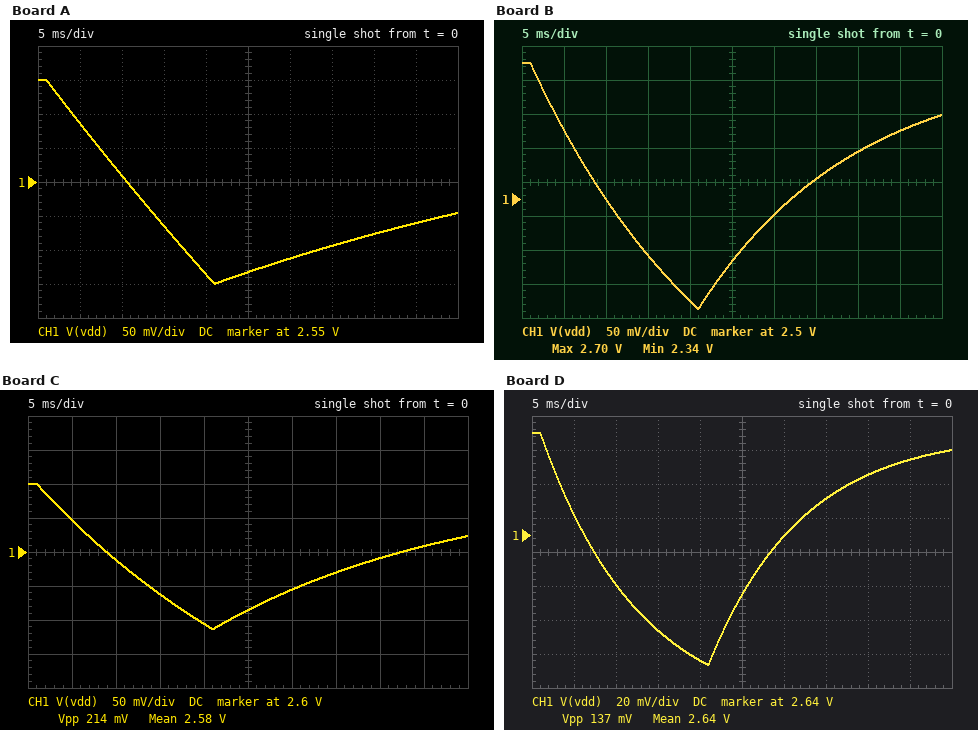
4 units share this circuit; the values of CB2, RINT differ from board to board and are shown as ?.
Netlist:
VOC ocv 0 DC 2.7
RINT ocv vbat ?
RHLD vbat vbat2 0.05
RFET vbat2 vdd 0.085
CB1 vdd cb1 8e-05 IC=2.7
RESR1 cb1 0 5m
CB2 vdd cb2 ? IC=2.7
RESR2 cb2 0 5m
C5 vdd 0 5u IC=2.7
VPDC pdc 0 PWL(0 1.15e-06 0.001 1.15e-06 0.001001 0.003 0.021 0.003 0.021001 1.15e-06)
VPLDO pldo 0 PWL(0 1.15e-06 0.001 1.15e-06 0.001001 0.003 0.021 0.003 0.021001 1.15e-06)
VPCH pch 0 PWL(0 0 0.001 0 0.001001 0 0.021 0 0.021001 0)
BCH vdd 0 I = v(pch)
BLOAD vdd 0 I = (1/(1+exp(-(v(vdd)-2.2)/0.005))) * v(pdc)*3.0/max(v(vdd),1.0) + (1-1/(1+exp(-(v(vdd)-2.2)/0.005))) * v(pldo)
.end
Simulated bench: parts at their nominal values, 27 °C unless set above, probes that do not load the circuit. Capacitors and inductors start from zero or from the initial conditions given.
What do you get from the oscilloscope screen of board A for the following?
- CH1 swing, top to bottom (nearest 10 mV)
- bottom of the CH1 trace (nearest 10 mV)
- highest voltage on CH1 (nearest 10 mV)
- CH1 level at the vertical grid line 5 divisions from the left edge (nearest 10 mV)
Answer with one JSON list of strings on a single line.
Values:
["300 mV", "2.40 V", "2.70 V", "2.42 V"]
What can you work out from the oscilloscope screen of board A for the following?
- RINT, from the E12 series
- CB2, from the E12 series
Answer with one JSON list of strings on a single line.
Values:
["330 Ω", "120 µF"]
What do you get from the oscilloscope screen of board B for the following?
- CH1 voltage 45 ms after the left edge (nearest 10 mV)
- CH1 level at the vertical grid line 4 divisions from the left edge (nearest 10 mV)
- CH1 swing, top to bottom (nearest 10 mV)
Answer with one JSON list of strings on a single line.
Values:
["2.60 V", "2.35 V", "360 mV"]
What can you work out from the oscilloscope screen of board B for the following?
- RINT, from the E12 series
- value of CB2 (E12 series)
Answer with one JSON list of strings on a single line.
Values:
["150 Ω", "39 µF"]
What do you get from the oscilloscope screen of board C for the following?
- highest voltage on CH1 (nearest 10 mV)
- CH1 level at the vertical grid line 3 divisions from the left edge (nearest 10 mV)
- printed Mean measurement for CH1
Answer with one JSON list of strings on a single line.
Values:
["2.70 V", "2.54 V", "2.58 V"]
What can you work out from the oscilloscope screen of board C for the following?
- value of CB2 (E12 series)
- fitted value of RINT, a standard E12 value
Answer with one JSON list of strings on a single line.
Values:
["150 µF", "120 Ω"]
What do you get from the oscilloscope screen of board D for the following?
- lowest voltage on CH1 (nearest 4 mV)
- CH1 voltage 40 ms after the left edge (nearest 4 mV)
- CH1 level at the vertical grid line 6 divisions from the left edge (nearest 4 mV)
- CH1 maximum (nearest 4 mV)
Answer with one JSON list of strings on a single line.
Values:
["2.564 V", "2.676 V", "2.640 V", "2.700 V"]
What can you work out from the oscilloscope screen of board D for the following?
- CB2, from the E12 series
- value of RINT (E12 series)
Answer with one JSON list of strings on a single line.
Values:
["150 µF", "47 Ω"]
